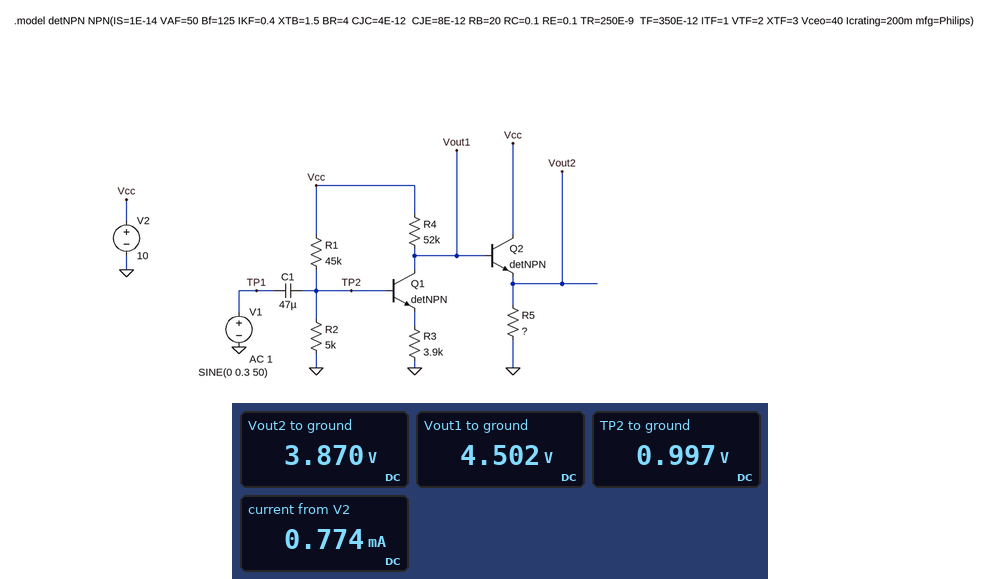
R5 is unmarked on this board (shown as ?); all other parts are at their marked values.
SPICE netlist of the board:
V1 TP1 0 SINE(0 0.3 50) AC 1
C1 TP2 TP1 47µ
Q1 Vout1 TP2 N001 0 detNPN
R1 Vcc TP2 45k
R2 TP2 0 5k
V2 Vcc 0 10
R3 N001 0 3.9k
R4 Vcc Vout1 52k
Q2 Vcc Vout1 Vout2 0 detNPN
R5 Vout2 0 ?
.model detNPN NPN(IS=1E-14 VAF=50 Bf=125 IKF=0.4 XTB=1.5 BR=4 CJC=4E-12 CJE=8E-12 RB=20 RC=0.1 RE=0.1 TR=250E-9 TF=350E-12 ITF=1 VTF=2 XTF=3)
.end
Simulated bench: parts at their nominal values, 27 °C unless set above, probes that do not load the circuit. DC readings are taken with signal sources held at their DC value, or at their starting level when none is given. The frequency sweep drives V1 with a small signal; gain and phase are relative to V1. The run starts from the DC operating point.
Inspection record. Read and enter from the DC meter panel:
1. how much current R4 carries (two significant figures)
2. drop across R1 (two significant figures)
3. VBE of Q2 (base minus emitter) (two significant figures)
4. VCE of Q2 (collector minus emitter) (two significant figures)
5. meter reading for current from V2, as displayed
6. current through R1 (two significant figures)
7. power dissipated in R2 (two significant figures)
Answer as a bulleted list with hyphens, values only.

- 110 µA
- 9.0 V
- 630 mV
- 6.1 V
- 0.774 mA
- 200 µA
- 200 µW
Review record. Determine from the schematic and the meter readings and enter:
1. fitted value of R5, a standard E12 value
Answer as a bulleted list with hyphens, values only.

- 8.2 kΩ
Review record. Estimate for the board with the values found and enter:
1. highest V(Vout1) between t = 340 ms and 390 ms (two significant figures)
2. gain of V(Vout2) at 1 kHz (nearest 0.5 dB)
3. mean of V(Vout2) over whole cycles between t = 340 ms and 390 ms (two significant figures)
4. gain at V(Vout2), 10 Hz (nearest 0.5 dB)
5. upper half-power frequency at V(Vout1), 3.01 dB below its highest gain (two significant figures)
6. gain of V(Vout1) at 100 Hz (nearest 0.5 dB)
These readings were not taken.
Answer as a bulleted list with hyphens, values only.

- 7.9 V
- 21.5 dB
- 3.8 V
- 21.5 dB
- 740 kHz
- 21.5 dB
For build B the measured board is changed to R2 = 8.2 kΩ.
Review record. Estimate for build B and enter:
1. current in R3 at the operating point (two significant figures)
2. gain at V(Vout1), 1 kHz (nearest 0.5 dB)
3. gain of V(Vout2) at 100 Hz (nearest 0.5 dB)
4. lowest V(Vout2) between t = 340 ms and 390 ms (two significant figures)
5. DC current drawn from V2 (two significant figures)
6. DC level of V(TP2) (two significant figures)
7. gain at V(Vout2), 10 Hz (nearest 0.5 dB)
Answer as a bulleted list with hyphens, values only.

- 200 µA
- -3.5 dB
- -4.0 dB
- 220 mV
- 400 µA
- 1.4 V
- -4.5 dB
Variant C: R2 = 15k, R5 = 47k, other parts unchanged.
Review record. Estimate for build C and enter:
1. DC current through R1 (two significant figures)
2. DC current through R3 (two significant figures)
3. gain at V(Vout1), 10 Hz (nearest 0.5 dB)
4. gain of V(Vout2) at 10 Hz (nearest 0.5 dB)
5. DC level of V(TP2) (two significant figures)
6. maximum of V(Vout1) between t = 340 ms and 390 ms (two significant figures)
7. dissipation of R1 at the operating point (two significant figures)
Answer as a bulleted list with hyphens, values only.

- 190 µA
- 250 µA
- -1.0 dB
- -1.5 dB
- 1.6 V
- 1.3 V
- 1.6 mW
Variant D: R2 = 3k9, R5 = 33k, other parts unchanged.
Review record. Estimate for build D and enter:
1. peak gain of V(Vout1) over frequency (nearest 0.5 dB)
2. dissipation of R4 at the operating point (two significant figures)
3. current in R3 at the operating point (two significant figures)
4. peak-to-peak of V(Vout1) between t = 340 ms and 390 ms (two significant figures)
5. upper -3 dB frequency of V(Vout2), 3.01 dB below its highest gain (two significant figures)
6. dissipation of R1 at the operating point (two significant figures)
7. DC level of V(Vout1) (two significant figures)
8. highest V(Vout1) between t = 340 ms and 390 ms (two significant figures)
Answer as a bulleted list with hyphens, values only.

- 21.5 dB
- 170 µW
- 56 µA
- 6.4 V
- 720 kHz
- 1.9 mW
- 7.0 V
- 9.8 V
